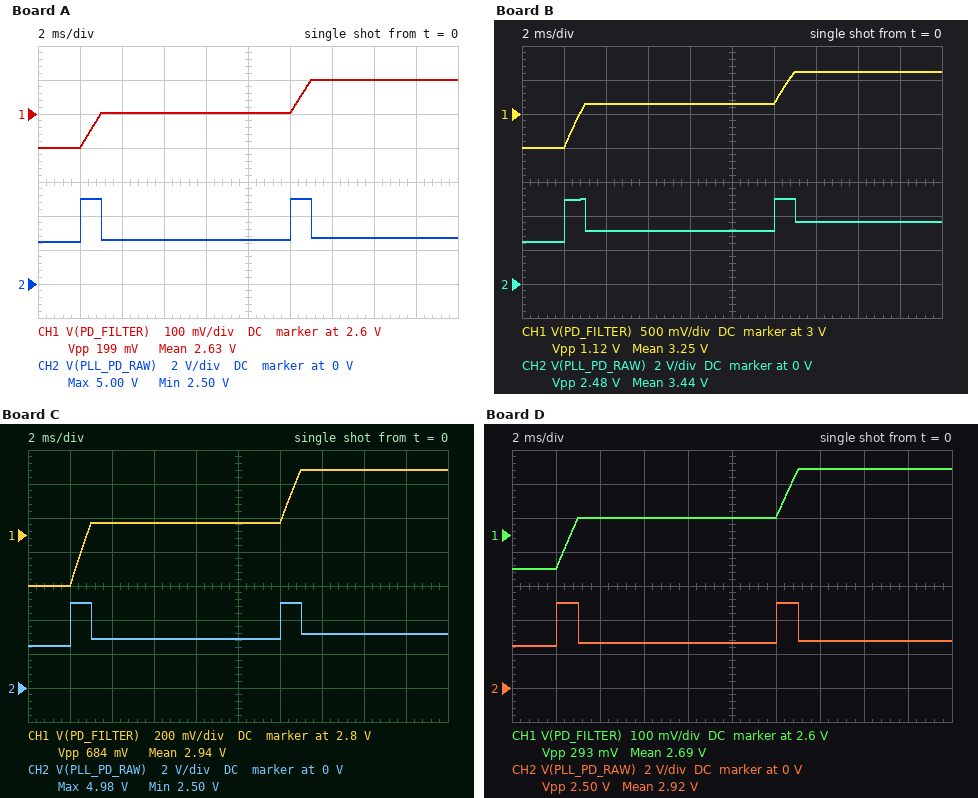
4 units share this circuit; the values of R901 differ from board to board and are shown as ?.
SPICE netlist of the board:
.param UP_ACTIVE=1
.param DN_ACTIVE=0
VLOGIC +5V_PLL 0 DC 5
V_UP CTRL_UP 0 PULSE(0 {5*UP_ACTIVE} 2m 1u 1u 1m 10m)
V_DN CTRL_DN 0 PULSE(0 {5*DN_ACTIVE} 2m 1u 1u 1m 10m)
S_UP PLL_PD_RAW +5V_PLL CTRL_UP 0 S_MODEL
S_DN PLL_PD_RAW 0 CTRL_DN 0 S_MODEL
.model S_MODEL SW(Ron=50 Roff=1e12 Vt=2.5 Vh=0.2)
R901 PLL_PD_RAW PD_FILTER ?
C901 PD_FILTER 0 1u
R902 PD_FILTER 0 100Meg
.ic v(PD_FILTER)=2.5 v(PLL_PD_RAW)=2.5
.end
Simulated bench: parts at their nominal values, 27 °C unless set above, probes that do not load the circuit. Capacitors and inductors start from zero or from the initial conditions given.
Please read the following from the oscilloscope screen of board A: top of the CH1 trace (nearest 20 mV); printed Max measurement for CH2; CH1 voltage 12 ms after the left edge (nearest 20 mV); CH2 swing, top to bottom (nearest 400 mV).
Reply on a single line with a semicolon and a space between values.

2.70 V; 5.00 V; 2.60 V; 2.4 V
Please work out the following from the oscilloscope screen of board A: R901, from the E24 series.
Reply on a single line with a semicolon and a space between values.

24 kΩ
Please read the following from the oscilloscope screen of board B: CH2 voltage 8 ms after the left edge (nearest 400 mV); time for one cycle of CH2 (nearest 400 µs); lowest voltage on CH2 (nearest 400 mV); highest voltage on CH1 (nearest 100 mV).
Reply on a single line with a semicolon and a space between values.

3.2 V; 10.0 ms; 2.4 V; 3.6 V
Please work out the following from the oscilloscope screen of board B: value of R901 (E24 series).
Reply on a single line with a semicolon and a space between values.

3.3 kΩ
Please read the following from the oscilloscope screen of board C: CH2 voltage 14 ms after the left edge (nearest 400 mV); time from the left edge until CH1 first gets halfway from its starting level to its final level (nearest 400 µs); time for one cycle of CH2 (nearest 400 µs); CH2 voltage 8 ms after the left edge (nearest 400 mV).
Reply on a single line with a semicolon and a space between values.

3.2 V; 2.8 ms; 10.0 ms; 2.8 V
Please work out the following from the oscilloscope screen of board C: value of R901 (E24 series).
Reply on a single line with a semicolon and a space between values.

6.2 kΩ
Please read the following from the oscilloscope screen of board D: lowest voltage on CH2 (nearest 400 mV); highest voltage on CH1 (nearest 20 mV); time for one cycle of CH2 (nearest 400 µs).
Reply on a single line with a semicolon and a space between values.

2.4 V; 2.80 V; 10.0 ms
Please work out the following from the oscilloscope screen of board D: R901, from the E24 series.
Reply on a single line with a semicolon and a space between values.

16 kΩ
